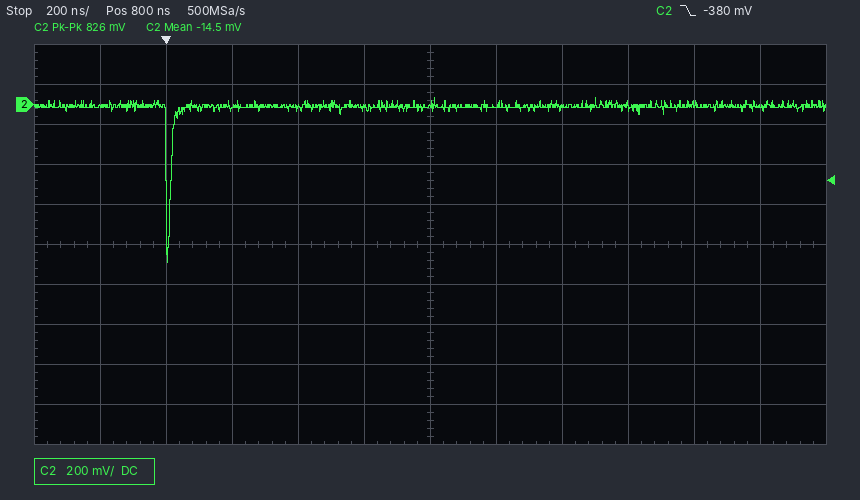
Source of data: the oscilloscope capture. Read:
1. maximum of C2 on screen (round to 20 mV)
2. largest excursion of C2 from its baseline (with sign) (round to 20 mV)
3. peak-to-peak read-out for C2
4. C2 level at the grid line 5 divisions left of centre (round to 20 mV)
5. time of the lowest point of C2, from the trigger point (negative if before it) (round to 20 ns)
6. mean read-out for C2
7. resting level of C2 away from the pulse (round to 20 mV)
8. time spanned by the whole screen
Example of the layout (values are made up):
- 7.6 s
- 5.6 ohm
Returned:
- 40 mV
- -780 mV
- 826 mV
- 0 mV
- 0 ns
- -14.5 mV
- 0 mV
- 2.4 µs
